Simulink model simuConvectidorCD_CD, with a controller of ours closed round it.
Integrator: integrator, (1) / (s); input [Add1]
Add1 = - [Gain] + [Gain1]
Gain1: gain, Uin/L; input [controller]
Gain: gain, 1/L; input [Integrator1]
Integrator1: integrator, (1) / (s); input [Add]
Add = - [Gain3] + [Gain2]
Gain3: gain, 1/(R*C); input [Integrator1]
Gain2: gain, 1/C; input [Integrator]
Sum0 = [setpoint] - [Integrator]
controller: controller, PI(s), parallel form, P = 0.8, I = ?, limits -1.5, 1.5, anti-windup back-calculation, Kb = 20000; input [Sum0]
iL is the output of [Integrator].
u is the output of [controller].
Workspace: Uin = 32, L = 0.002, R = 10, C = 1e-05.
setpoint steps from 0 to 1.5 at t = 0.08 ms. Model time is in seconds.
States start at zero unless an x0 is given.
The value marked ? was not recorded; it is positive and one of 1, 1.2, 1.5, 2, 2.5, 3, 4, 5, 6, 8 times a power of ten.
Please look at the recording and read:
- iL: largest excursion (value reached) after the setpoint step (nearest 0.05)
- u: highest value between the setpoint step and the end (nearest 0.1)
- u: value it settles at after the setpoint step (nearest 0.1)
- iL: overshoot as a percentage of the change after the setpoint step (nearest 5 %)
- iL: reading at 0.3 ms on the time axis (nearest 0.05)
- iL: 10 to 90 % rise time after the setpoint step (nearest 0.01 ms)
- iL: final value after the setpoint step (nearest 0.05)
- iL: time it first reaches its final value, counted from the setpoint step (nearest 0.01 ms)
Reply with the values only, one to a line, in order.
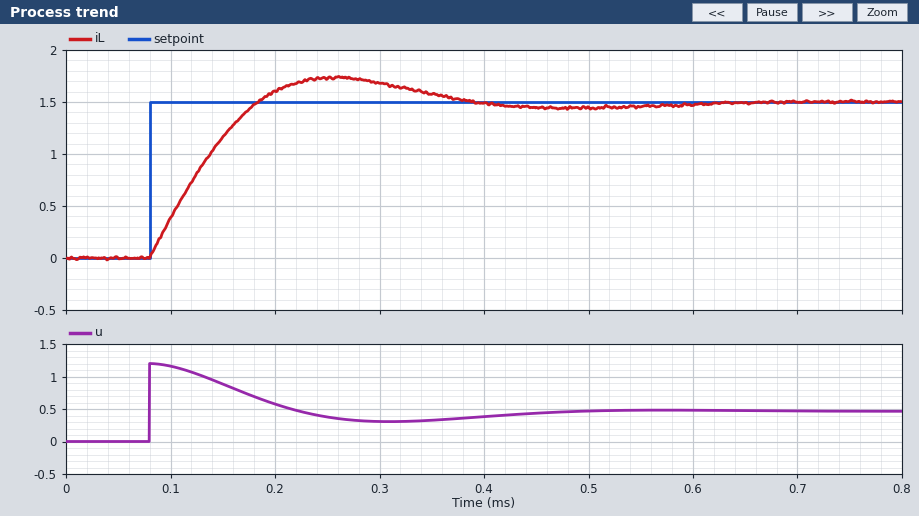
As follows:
1.75
1.2
0.5
15 %
1.70
0.08 ms
1.50
0.10 ms
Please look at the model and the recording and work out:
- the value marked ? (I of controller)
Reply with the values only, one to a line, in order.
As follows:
10000
